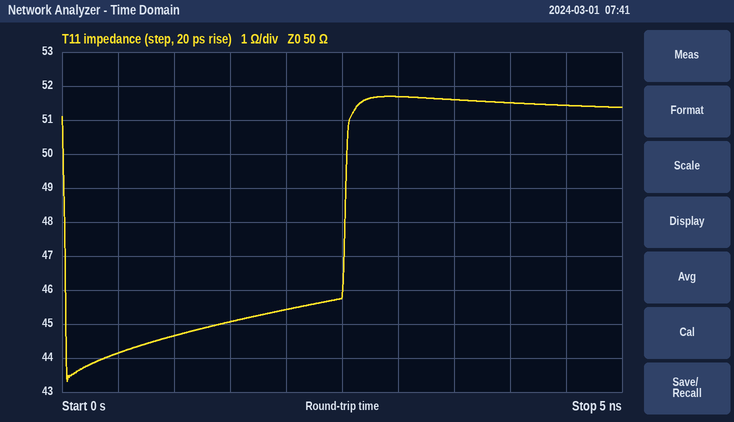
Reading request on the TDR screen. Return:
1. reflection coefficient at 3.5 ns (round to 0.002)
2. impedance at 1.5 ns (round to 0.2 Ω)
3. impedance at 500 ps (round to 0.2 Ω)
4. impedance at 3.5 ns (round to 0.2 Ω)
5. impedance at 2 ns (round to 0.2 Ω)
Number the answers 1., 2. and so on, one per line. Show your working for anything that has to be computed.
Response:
1. (51.6 − 50)/(51.6 + 50) ≈ +0.016
2. 45.0 Ω
3. 44.2 Ω
4. 51.6 Ω
5. 45.4 Ω
